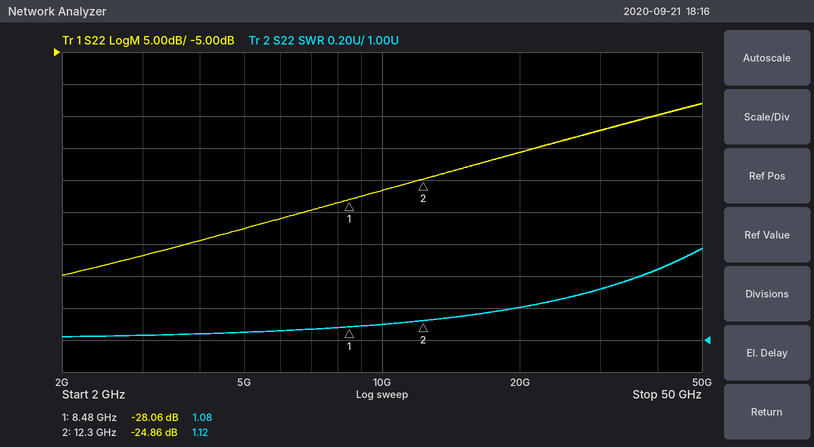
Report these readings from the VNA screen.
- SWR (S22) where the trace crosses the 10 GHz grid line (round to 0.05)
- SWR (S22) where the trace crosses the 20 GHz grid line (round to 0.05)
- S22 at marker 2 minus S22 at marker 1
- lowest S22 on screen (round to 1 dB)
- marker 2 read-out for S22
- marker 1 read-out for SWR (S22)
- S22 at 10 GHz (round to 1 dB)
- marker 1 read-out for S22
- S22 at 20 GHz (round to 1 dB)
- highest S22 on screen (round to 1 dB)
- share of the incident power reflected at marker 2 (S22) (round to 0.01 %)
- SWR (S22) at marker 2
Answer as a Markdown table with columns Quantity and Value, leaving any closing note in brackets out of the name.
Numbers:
| Quantity | Value |
|---|---|
| SWR (S22) where the trace crosses the 10 GHz grid line | 1.10 |
| SWR (S22) where the trace crosses the 20 GHz grid line | 1.20 |
| S22 at marker 2 minus S22 at marker 1 | 3.20 dB |
| lowest S22 on screen | -40 dB |
| marker 2 read-out for S22 | -24.86 dB |
| marker 1 read-out for SWR | 1.08 |
| S22 at 10 GHz | -27 dB |
| marker 1 read-out for S22 | -28.06 dB |
| S22 at 20 GHz | -21 dB |
| highest S22 on screen | -13 dB |
| share of the incident power reflected at marker 2 (S22) | 0.33 % |
| SWR (S22) at marker 2 | 1.12 |
